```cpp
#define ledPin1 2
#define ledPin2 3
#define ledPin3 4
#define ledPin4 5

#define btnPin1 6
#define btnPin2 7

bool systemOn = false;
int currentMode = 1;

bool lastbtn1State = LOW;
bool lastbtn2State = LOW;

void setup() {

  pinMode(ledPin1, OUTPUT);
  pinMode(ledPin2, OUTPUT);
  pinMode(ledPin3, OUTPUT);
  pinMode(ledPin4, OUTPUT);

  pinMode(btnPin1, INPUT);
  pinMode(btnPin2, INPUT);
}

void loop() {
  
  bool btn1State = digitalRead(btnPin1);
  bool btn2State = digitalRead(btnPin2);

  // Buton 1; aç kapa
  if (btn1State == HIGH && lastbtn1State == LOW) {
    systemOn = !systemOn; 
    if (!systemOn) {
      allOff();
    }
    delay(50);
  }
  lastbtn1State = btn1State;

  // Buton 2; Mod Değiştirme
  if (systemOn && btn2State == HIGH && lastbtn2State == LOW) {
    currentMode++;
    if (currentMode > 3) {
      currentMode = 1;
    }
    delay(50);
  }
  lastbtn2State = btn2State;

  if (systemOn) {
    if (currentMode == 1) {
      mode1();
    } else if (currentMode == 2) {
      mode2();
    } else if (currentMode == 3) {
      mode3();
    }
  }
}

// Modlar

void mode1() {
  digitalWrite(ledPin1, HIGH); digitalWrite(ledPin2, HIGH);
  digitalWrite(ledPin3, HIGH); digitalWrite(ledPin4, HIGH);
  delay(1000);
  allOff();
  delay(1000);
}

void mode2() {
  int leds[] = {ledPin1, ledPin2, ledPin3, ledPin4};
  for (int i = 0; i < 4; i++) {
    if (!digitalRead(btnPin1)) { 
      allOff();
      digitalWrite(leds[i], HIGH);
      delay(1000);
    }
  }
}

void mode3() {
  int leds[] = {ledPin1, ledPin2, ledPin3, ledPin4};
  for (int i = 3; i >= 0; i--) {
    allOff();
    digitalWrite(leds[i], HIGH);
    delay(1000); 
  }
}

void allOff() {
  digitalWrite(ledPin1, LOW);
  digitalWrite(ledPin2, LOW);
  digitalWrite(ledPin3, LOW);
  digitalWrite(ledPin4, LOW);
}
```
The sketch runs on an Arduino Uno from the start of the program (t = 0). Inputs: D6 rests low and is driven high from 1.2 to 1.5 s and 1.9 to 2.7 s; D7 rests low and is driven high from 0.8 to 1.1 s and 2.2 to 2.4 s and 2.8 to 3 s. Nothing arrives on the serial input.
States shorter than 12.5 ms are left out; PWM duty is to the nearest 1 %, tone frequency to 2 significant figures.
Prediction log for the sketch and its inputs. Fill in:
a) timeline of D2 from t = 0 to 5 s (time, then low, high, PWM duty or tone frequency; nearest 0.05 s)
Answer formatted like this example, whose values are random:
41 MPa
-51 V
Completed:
0 s low; 1.25 s high; 2.25 s low; 3.25 s high; 4.25 s low
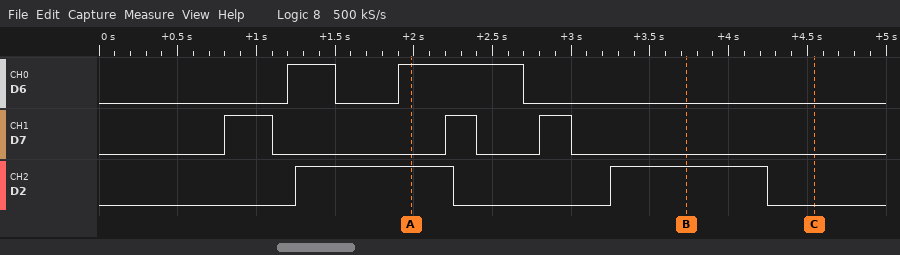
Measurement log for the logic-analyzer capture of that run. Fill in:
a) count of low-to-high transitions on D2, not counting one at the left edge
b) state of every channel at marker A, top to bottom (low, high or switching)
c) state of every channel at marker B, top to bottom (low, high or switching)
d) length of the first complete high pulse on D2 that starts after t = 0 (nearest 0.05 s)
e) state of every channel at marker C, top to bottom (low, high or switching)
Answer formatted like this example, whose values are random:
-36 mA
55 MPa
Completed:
2
D6 high, D7 low, D2 high
D6 low, D7 low, D2 high
1.00 s
D6 low, D7 low, D2 low
